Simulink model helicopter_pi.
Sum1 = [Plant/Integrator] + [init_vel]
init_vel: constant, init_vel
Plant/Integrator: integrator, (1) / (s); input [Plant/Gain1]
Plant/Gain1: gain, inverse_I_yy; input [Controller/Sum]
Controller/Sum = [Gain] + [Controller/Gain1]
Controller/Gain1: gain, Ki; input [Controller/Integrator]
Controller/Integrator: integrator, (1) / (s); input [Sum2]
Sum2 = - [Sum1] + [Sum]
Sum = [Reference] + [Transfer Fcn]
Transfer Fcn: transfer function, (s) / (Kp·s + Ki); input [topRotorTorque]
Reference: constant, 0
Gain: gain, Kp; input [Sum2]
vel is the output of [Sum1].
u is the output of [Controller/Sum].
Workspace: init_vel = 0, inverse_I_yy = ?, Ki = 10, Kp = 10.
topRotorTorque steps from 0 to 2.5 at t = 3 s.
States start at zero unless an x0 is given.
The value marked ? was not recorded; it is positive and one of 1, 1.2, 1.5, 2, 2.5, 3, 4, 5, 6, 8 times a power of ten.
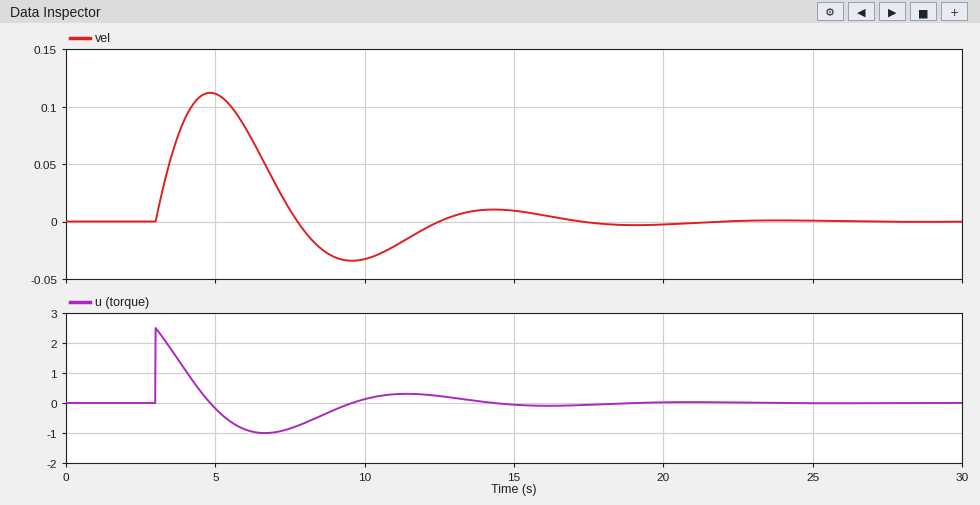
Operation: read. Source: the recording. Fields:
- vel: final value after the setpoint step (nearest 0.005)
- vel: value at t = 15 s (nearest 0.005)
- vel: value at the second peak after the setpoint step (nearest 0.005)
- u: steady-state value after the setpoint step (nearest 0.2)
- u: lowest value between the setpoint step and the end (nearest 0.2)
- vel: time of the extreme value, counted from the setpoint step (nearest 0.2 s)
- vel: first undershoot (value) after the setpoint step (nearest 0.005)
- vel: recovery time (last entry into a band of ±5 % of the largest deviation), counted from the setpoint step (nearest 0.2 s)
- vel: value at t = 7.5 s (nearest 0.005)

0.000
0.010
0.010
0.0
-1.0
1.8 s
-0.035
13.0 s
0.010
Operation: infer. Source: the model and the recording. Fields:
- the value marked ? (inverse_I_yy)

0.05
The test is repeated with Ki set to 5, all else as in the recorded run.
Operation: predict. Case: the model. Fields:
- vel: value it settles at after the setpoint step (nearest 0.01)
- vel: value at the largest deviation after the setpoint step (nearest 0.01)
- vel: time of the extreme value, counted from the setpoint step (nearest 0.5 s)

0.00
0.14
2.5 s
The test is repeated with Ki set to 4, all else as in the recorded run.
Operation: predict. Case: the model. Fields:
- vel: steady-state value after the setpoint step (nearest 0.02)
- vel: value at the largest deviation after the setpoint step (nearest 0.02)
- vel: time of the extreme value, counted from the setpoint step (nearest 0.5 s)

0.00
0.14
2.5 s
